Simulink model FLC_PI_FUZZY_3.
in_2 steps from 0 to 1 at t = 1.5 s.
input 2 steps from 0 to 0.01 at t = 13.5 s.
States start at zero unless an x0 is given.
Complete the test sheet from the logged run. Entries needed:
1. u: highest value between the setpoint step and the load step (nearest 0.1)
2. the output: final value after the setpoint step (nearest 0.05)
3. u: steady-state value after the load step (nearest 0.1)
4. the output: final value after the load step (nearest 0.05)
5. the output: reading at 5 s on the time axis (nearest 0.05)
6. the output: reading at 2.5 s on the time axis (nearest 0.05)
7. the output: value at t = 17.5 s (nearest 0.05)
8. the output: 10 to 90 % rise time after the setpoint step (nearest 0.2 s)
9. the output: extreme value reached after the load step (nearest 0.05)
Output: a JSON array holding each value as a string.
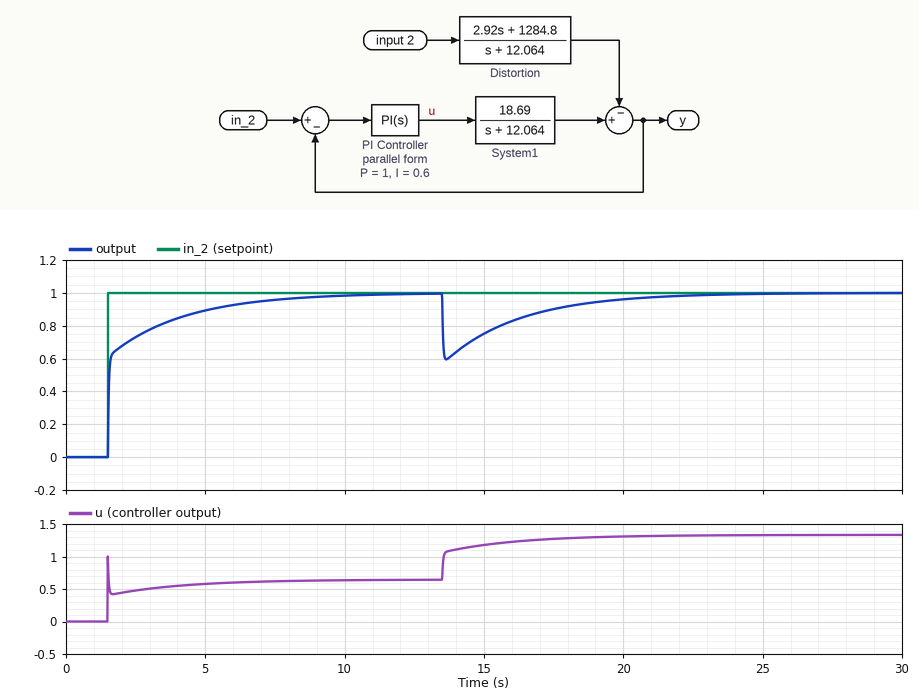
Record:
["1.0", "1.00", "1.3", "1.00", "0.90", "0.75", "0.90", "3.6 s", "0.60"]
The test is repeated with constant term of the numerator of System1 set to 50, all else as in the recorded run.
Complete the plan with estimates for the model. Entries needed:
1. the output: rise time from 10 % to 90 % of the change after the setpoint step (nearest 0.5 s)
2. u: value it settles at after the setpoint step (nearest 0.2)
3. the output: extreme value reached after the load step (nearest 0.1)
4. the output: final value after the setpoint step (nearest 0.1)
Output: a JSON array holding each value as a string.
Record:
["1.5 s", "0.2", "0.8", "1.0"]
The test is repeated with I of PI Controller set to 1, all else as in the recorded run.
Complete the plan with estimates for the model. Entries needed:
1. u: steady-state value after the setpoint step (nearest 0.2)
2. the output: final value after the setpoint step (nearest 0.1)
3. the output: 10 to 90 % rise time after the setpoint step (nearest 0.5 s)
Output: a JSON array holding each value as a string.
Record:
["0.6", "1.0", "2.0 s"]
